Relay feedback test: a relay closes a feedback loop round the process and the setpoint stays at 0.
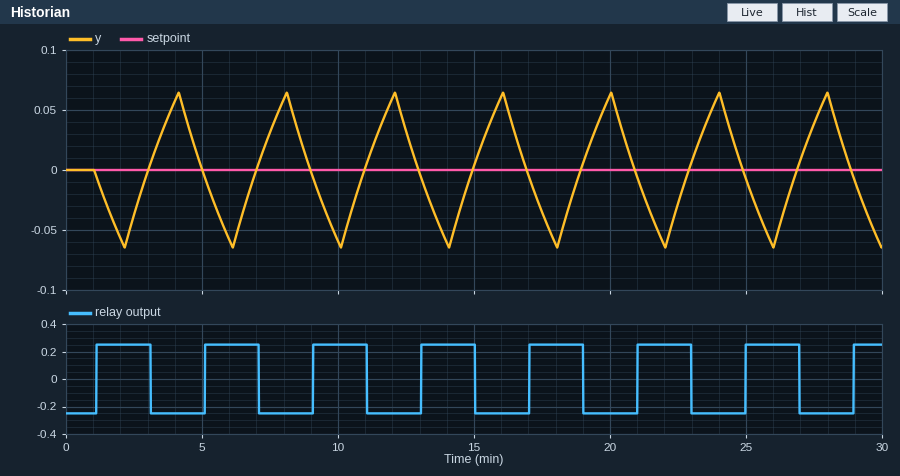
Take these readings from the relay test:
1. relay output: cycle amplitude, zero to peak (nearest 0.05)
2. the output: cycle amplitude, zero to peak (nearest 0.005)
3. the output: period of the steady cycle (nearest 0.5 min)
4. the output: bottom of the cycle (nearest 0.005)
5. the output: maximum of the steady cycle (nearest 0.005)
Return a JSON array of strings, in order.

["0.25", "0.065", "4.0 min", "-0.065", "0.065"]
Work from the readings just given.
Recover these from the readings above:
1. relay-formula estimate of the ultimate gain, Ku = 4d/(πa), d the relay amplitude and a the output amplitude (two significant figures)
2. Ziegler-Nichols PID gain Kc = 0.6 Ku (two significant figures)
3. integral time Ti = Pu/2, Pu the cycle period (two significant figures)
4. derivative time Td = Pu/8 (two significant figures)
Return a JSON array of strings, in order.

["4.9", "2.9", "2.0 min", "0.50 min"]
